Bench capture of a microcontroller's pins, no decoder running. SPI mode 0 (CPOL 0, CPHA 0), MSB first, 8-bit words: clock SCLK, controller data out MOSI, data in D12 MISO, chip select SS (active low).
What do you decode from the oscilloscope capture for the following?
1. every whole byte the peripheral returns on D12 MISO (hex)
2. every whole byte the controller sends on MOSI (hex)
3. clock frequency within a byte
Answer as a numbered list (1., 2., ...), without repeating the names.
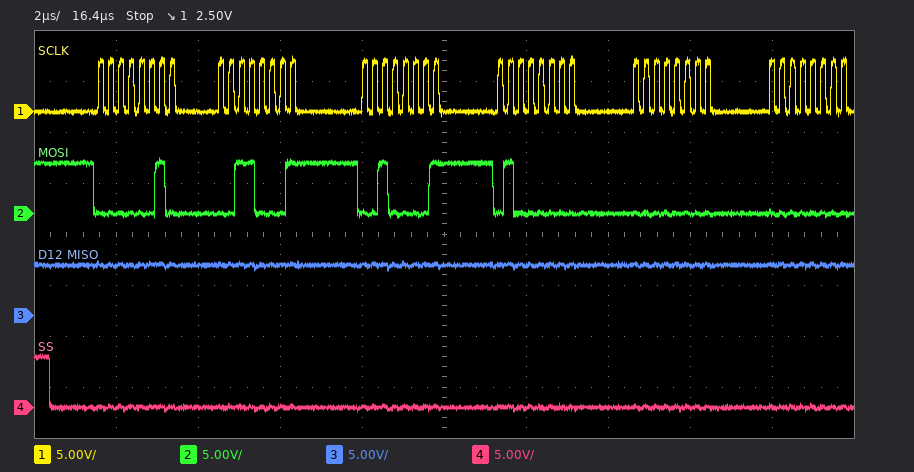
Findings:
1. FF FF FF FF FF FF
2. 02 31 21 40 00 00
3. 4 MHz
